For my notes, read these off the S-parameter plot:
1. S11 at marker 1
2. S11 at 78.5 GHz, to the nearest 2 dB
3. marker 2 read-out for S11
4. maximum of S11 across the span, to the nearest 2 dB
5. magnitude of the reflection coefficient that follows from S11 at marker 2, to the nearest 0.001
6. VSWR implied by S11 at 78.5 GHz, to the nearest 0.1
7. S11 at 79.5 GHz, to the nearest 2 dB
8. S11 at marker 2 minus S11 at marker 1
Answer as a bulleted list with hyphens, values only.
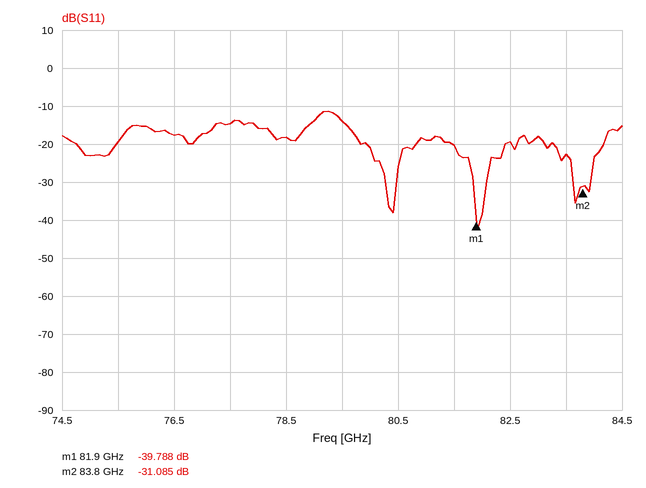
- -39.788 dB
- -18 dB
- -31.085 dB
- -12 dB
- 0.028
- 1.3
- -14 dB
- 8.703 dB
